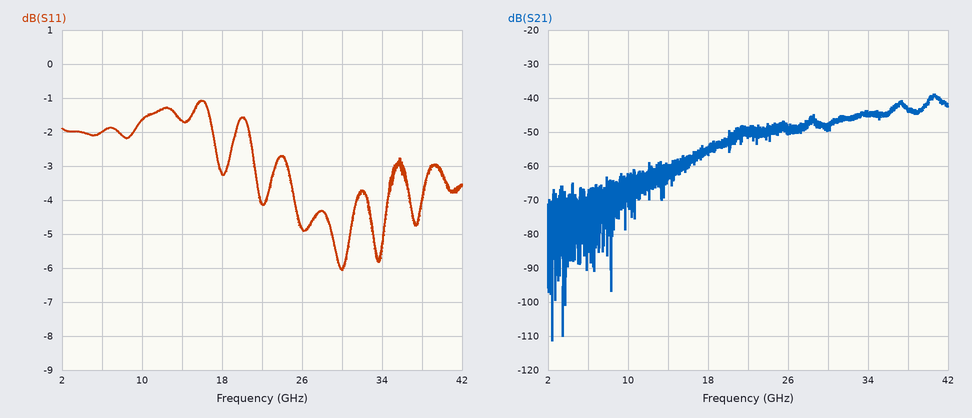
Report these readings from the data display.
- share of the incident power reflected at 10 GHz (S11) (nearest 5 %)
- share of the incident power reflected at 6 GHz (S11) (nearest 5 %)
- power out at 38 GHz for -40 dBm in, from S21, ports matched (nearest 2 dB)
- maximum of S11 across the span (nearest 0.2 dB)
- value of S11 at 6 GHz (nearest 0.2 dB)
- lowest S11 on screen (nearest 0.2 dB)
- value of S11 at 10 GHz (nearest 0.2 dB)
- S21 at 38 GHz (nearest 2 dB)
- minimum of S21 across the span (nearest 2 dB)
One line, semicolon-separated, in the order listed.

70 %; 65 %; -84 dBm; -1.0 dB; -2.0 dB; -6.0 dB; -1.6 dB; -44 dB; -112 dB
